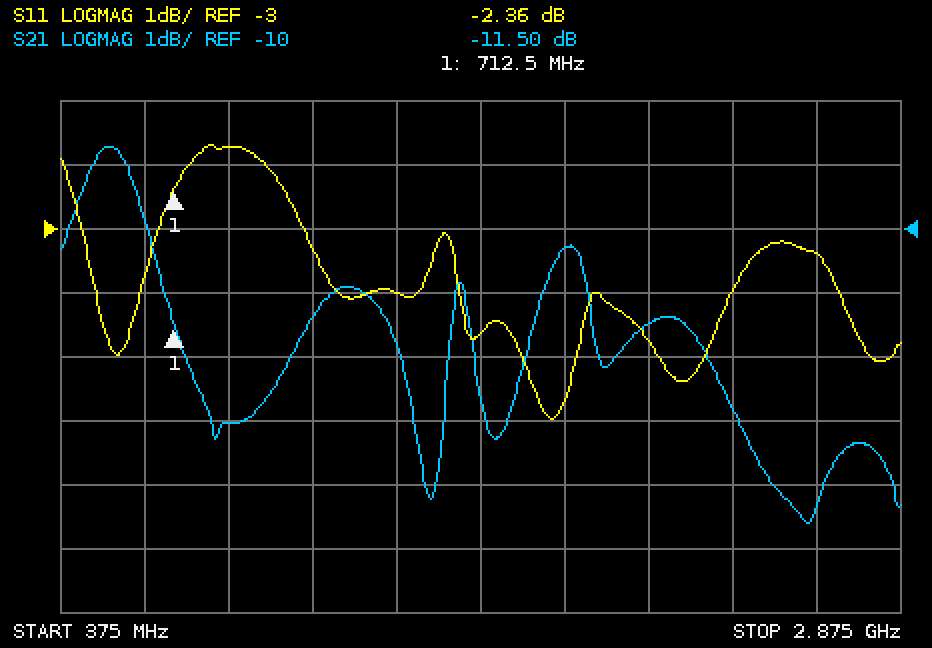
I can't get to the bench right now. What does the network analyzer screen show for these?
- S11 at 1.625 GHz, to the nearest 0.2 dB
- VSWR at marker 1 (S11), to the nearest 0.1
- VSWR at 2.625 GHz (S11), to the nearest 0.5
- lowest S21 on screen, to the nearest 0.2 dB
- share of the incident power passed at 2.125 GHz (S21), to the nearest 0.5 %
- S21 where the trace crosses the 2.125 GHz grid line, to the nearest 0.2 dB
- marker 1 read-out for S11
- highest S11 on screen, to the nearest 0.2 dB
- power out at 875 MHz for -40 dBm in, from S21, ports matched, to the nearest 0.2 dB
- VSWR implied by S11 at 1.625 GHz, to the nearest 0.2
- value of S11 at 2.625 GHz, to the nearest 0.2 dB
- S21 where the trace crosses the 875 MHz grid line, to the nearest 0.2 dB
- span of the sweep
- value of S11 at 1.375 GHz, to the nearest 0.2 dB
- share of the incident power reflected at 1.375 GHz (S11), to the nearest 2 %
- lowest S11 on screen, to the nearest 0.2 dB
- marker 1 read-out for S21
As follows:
-4.6 dB
7.4
5.0
-14.6 dB
7.0 %
-11.4 dB
-2.36 dB
-1.6 dB
-53.0 dBm
3.8
-3.4 dB
-13.0 dB
2.5 GHz
-4.0 dB
40 %
-6.0 dB
-11.50 dB
